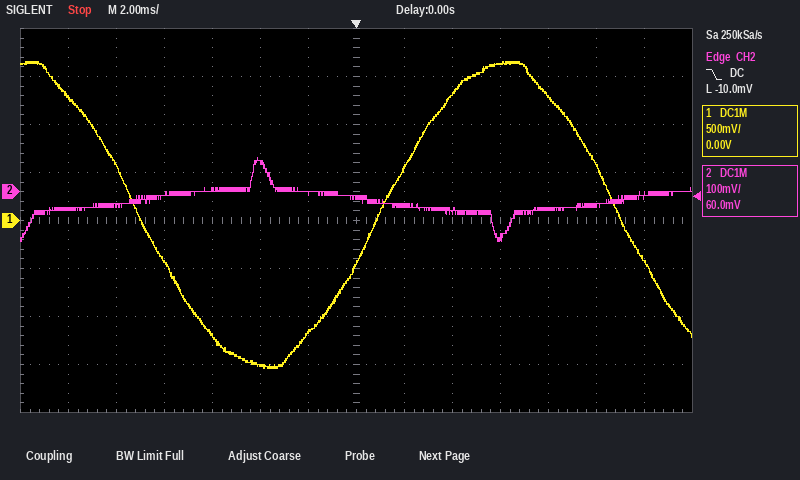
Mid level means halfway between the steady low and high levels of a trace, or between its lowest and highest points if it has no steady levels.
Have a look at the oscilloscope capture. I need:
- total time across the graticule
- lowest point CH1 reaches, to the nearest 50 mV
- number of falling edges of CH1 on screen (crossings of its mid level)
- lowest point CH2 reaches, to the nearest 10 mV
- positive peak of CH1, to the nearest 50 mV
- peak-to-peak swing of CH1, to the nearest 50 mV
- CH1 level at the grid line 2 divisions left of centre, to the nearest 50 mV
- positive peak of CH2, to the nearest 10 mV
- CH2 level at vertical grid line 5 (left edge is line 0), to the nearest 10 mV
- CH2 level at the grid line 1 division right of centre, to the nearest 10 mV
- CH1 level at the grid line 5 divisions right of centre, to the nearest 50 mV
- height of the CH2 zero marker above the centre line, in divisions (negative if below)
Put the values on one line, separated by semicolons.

28 ms; -1.55 V; 2; -100 mV; 1.65 V; 3.20 V; -1.50 V; 70 mV; 60 mV; -30 mV; 600 mV; +0.6 div
